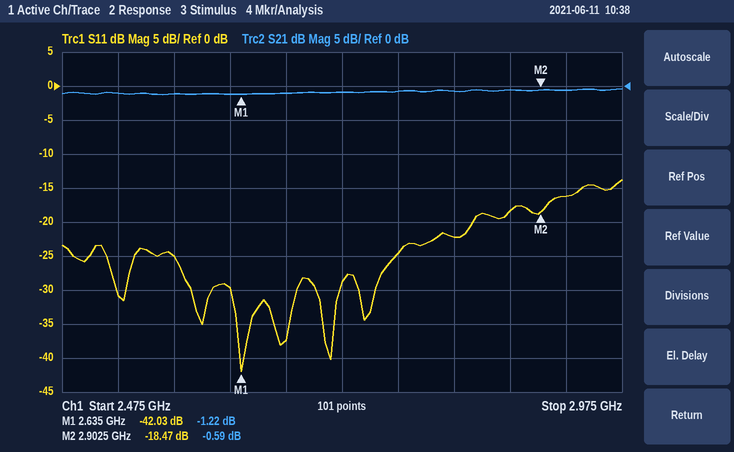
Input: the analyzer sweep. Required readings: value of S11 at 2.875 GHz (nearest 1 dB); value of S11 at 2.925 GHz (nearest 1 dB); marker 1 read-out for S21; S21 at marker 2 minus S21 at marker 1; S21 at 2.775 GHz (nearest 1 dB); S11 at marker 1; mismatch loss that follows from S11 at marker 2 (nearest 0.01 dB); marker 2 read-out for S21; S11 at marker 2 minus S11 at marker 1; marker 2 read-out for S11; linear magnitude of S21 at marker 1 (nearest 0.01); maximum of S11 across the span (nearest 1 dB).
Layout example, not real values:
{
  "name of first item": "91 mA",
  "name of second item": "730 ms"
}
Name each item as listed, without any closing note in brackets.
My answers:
{
  "value of S11 at 2.875 GHz": "-18 dB",
  "value of S11 at 2.925 GHz": "-16 dB",
  "marker 1 read-out for S21": "-1.22 dB",
  "S21 at marker 2 minus S21 at marker 1": "0.63 dB",
  "S21 at 2.775 GHz": "-1 dB",
  "S11 at marker 1": "-42.03 dB",
  "mismatch loss that follows from S11 at marker 2": "0.06 dB",
  "marker 2 read-out for S21": "-0.59 dB",
  "S11 at marker 2 minus S11 at marker 1": "23.56 dB",
  "marker 2 read-out for S11": "-18.47 dB",
  "linear magnitude of S21 at marker 1": "0.87",
  "maximum of S11 across the span": "-14 dB"
}
